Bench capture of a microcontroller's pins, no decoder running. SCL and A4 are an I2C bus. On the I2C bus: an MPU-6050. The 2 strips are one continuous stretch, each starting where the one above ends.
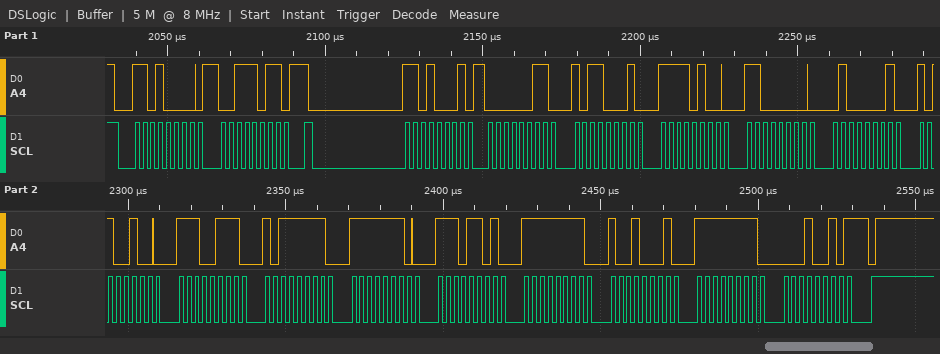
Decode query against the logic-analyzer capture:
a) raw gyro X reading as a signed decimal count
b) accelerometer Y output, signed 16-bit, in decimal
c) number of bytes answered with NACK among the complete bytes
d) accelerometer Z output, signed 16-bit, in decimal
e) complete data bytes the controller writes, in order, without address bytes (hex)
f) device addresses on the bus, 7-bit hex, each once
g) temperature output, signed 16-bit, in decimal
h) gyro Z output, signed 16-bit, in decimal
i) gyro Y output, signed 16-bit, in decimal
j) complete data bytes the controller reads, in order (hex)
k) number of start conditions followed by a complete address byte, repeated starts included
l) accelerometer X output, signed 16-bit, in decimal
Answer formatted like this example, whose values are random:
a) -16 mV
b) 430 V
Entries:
a) -275
b) -2880
c) 1
d) 16804
e) 3B
f) 0x68
g) -6209
h) -238
i) -111
j) 03 B1 F4 C0 41 A4 E7 BF FE ED FF 91 FF 12
k) 2
l) 945
